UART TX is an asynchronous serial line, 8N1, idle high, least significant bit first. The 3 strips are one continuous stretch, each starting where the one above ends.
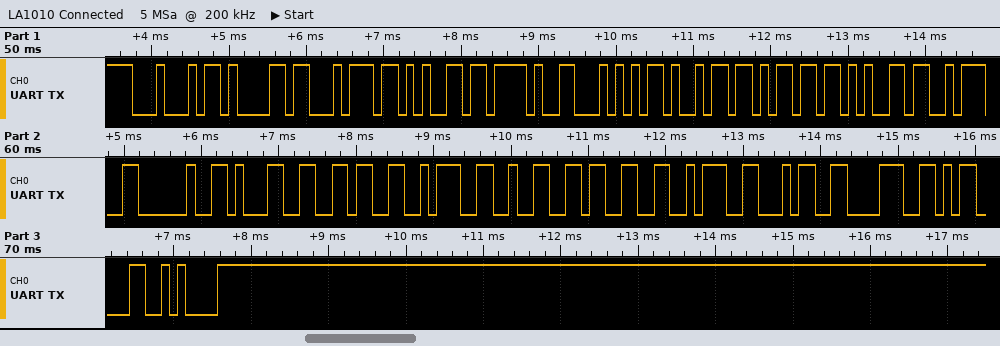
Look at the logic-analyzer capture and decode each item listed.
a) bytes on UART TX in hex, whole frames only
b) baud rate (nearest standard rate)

0x44 0x61 0x74 0x65 0x2F 0x54 0x69 0x6D 0x65 0x3A 0x20 0x31 0x36 0x3A 0x32 0x33 0x3A 0x34 0x38 0x0D 0x0A
9600 baud
